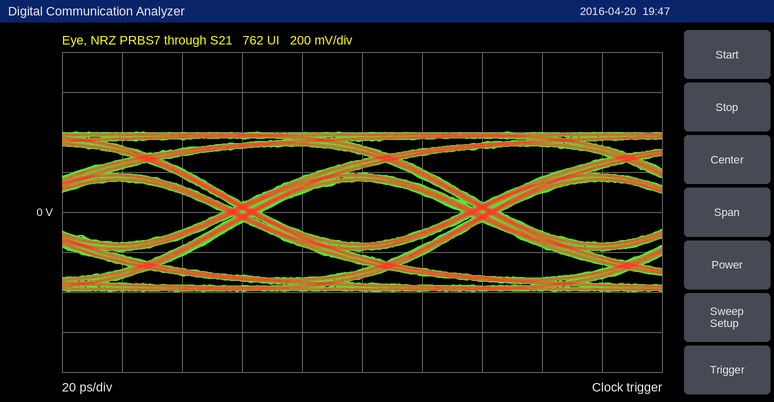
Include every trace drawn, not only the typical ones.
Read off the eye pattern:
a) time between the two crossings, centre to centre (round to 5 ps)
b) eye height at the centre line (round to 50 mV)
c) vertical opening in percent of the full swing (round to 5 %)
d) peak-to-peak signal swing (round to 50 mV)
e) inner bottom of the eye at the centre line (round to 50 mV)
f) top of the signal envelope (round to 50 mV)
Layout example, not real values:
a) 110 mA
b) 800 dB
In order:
a) 80 ps
b) 300 mV
c) 40 %
d) 800 mV
e) -150 mV
f) 400 mV
